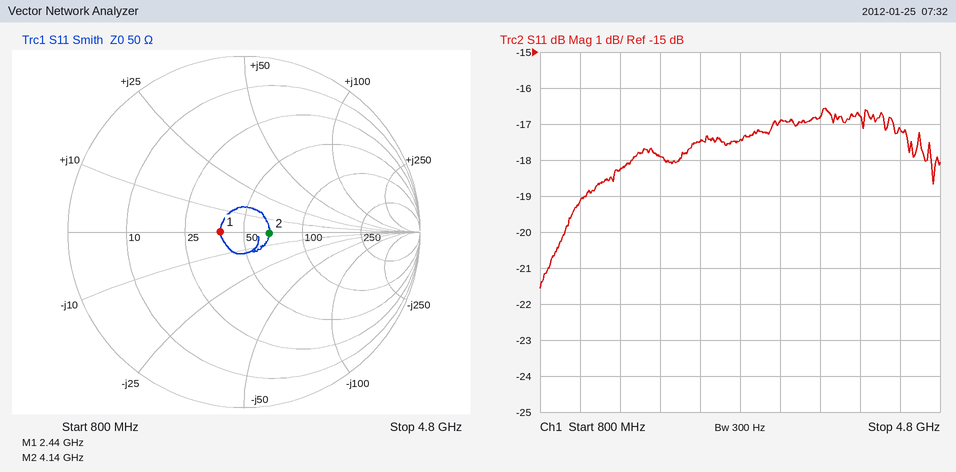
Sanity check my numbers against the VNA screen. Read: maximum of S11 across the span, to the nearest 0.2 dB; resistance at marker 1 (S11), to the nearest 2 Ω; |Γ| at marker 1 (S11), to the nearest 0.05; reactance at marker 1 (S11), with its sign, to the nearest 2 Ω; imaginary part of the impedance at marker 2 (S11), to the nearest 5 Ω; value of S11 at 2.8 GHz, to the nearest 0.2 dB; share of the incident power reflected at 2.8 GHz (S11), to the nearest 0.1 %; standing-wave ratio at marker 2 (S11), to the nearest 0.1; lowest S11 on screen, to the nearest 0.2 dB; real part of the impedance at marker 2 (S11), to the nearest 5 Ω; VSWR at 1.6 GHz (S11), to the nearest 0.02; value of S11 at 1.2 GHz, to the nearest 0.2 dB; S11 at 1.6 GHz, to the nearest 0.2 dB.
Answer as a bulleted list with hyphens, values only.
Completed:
- -16.6 dB
- 38 Ω
- 0.15
- 0 Ω
- 0 Ω
- -17.4 dB
- 1.8 %
- 1.3
- -21.6 dB
- 65 Ω
- 1.28
- -19.2 dB
- -18.2 dB
